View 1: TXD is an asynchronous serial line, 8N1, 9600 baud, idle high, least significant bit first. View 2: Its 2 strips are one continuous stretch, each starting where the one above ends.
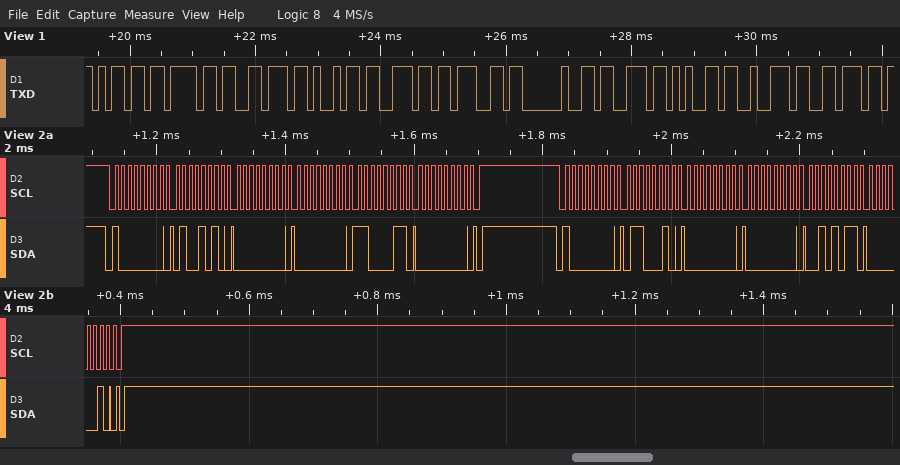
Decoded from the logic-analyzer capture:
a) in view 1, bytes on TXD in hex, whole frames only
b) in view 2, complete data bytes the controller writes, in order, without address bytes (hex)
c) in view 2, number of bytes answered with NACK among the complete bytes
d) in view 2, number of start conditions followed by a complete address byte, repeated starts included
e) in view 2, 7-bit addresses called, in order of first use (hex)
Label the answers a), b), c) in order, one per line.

a) 6D 6F 76 69 6E 67 20 73 65 72 76
b) 4A 00 00 C3 00 62 00 00 2B 02
c) 0
d) 2
e) 0x40
